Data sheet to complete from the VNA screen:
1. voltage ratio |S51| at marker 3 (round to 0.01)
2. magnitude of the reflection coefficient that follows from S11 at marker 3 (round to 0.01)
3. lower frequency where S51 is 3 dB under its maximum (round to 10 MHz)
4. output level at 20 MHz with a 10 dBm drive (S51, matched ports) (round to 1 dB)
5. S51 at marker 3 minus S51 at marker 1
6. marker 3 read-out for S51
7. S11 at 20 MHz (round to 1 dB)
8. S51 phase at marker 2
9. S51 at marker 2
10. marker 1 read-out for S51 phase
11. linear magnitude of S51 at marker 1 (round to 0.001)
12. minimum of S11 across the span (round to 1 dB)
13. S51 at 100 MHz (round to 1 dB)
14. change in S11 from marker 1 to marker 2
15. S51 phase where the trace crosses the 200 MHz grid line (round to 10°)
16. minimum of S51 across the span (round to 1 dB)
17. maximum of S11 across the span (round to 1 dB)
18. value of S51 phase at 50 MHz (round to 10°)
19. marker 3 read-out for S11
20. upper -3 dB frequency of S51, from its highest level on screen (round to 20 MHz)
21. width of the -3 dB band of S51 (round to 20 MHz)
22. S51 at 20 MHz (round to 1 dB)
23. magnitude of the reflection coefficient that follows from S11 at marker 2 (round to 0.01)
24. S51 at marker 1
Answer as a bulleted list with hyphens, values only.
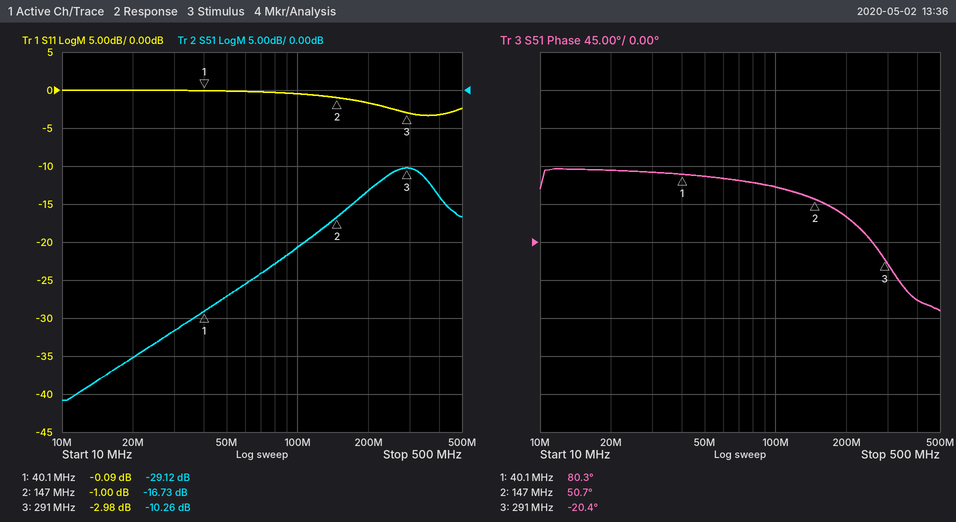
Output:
- 0.31
- 0.71
- 200 MHz
- -25 dBm
- 18.86 dB
- -10.26 dB
- 0 dB
- 50.7°
- -16.73 dB
- 80.3°
- 0.035
- -3 dB
- -21 dB
- -0.91 dB
- 30°
- -41 dB
- 0 dB
- 80°
- -2.98 dB
- 380 MHz
- 180 MHz
- -35 dB
- 0.89
- -29.12 dB
